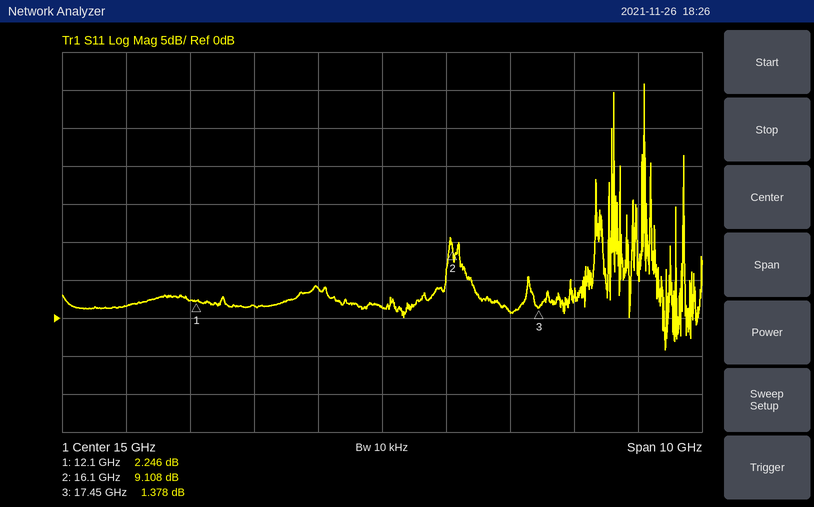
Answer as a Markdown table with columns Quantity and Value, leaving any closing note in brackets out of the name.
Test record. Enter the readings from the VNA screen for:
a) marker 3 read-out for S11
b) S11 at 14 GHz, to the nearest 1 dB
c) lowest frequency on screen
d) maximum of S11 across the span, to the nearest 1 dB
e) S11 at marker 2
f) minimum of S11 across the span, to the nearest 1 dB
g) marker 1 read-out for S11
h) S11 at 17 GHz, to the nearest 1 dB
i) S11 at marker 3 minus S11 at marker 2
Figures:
| Quantity | Value |
|---|---|
| marker 3 read-out for S11 | 1.378 dB |
| S11 at 14 GHz, to the nearest 1 dB | 4 dB |
| lowest frequency on screen | 10 GHz |
| maximum of S11 across the span, to the nearest 1 dB | 31 dB |
| S11 at marker 2 | 9.108 dB |
| minimum of S11 across the span, to the nearest 1 dB | -4 dB |
| marker 1 read-out for S11 | 2.246 dB |
| S11 at 17 GHz, to the nearest 1 dB | 1 dB |
| S11 at marker 3 minus S11 at marker 2 | -7.730 dB |
